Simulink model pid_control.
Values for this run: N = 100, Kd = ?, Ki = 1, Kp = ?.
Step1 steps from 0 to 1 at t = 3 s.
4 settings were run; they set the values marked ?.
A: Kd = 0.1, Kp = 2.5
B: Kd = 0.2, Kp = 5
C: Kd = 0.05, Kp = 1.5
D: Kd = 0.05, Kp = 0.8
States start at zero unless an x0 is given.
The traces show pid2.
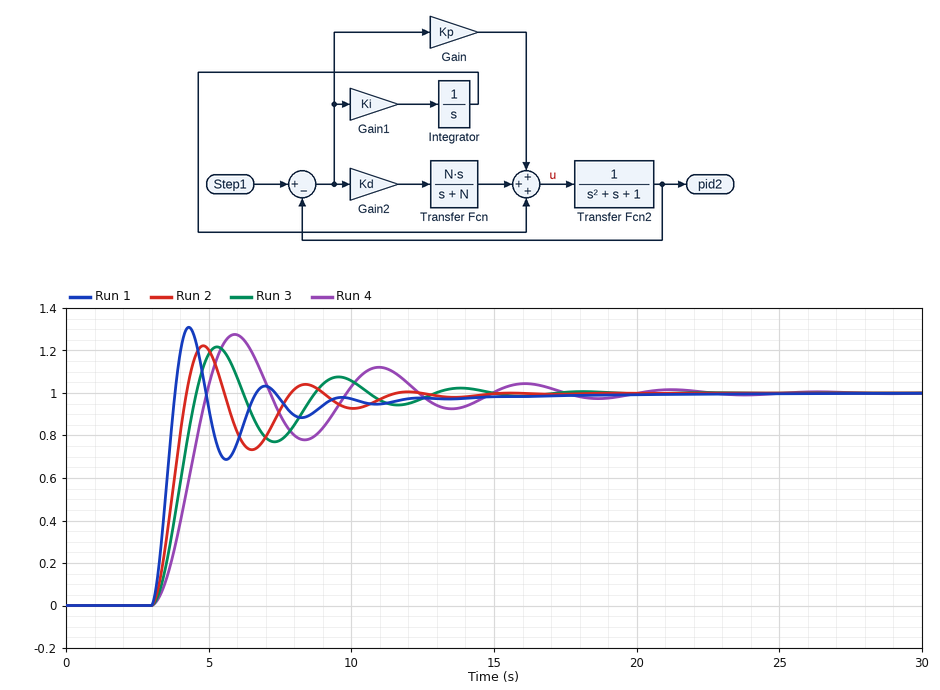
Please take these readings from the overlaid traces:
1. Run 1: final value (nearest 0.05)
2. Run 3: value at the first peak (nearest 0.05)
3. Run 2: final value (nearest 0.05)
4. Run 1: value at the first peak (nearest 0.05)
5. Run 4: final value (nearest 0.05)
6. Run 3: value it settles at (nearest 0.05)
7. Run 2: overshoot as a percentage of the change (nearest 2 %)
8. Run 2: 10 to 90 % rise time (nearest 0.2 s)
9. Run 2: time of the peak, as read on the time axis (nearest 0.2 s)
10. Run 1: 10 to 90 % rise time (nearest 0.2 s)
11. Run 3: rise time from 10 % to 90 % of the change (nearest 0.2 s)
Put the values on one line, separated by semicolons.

1.00; 1.20; 1.00; 1.30; 1.00; 1.00; 22 %; 0.8 s; 4.8 s; 0.6 s; 1.0 s
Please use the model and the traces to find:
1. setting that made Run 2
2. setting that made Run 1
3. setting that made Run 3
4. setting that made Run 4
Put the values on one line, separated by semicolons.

A; B; C; D
